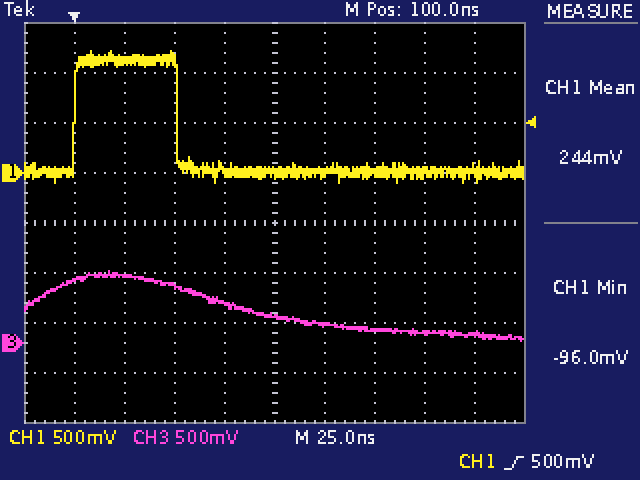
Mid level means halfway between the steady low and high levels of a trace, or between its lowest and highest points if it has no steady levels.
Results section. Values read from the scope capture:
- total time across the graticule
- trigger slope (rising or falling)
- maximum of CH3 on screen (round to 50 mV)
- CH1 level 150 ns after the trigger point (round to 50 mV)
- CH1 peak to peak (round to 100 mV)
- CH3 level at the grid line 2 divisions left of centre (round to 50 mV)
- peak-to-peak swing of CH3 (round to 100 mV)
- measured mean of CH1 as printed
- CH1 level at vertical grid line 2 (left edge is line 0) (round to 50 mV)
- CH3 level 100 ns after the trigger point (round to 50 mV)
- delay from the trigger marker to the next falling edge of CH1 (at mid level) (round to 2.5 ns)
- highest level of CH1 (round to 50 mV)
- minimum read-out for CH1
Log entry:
250 ns
rising
700 mV
0 mV
1.30 V
550 mV
700 mV
244 mV
1.10 V
250 mV
52.5 ns
1.20 V
-96.0 mV
